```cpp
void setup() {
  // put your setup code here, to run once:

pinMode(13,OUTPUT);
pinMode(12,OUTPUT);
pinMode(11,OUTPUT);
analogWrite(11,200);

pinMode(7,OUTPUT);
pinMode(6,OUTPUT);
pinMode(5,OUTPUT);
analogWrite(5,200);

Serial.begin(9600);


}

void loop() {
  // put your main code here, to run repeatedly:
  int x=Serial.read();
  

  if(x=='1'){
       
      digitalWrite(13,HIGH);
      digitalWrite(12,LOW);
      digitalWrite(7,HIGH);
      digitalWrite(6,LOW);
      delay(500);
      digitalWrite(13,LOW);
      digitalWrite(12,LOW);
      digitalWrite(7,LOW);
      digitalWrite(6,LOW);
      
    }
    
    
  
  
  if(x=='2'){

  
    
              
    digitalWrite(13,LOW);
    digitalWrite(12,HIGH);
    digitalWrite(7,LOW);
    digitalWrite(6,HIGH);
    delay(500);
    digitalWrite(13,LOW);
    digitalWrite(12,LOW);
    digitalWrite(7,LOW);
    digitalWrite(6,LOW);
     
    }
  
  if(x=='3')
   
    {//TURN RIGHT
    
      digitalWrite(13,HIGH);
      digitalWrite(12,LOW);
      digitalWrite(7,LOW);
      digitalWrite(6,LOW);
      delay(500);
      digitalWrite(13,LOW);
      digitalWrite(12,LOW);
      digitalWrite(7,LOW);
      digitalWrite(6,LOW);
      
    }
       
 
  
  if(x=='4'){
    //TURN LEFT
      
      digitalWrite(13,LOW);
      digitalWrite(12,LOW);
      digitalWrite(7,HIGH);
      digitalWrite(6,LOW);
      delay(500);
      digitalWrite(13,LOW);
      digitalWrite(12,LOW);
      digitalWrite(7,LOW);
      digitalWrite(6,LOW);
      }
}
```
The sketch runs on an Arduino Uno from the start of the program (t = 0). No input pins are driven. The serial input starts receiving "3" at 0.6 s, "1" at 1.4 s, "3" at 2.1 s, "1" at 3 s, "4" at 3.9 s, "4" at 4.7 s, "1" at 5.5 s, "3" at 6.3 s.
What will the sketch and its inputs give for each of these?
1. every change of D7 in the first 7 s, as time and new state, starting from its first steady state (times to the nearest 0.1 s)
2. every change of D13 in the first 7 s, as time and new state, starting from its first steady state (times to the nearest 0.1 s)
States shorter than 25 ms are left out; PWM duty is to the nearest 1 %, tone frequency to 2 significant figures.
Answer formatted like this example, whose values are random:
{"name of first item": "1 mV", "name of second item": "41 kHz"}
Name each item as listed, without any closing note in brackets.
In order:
{"every change of D7 in the first 7 s, as time and new state, starting from its first steady state": "0 s low; 1.4 s high; 1.9 s low; 3 s high; 3.5 s low; 3.9 s high; 4.4 s low; 4.7 s high; 5.2 s low; 5.5 s high; 6 s low", "every change of D13 in the first 7 s, as time and new state, starting from its first steady state": "0 s low; 0.6 s high; 1.1 s low; 1.4 s high; 1.9 s low; 2.1 s high; 2.6 s low; 3 s high; 3.5 s low; 5.5 s high; 6 s low; 6.3 s high; 6.8 s low"}
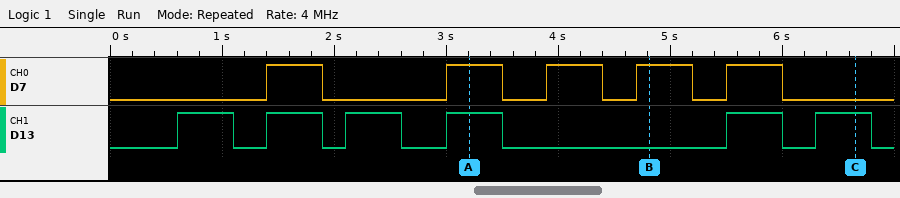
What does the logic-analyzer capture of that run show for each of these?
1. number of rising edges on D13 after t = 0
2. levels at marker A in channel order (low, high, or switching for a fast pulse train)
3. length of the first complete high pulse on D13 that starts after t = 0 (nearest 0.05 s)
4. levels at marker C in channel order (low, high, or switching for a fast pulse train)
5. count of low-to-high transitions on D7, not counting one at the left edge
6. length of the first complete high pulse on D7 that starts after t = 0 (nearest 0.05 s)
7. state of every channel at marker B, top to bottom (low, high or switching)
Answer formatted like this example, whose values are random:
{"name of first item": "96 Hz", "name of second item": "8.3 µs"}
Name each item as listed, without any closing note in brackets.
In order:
{"number of rising edges on D13 after t = 0": "6", "levels at marker A in channel order": "D7 high, D13 high", "length of the first complete high pulse on D13 that starts after t = 0": "0.50 s", "levels at marker C in channel order": "D7 low, D13 high", "count of low-to-high transitions on D7, not counting one at the left edge": "5", "length of the first complete high pulse on D7 that starts after t = 0": "0.50 s", "state of every channel at marker B, top to bottom": "D7 high, D13 low"}
